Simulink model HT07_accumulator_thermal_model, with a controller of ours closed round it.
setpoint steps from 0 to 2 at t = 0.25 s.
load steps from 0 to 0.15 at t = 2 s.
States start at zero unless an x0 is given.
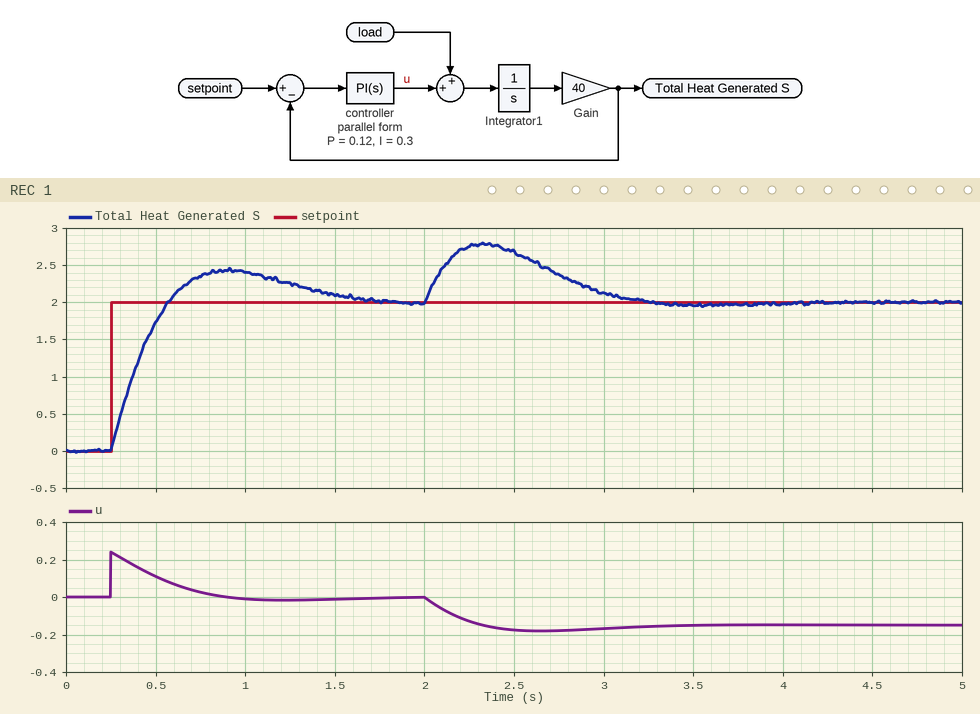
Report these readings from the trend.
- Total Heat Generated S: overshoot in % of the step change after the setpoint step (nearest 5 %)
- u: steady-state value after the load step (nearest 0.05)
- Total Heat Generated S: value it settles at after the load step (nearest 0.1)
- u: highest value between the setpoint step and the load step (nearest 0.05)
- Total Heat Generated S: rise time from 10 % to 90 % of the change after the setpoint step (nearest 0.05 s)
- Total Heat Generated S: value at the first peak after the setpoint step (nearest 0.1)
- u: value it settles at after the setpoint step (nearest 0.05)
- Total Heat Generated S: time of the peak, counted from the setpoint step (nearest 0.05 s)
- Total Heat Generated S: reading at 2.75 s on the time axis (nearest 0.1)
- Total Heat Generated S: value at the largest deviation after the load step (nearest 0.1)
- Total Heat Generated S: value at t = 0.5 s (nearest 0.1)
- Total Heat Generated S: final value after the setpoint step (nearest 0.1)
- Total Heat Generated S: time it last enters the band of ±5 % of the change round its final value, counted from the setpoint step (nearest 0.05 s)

20 %
-0.15
2.0
0.25
0.25 s
2.4
0.00
0.65 s
2.4
2.8
1.7
2.0
1.25 s
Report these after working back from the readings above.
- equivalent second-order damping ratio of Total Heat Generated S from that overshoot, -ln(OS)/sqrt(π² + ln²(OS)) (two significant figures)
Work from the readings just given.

0.46
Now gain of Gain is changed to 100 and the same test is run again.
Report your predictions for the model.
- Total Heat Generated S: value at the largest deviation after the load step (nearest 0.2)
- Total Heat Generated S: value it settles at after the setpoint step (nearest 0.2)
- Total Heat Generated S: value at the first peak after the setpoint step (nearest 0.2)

3.0
2.0
2.2
